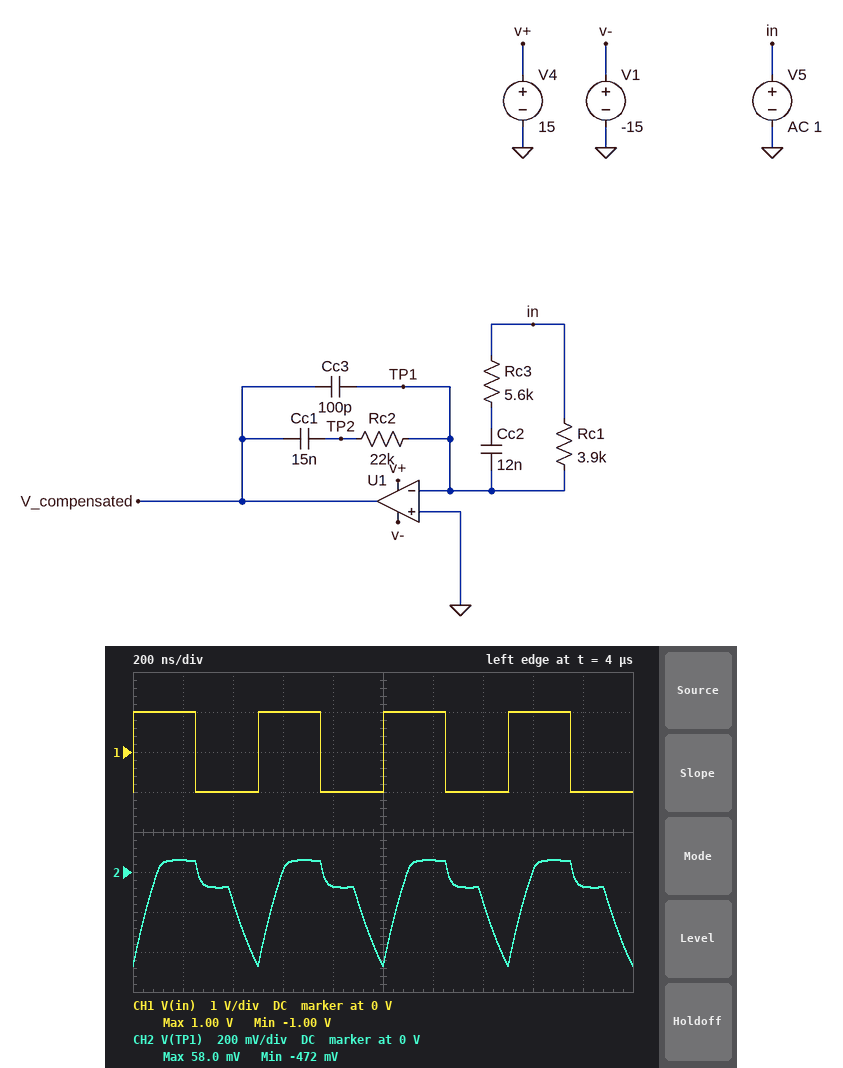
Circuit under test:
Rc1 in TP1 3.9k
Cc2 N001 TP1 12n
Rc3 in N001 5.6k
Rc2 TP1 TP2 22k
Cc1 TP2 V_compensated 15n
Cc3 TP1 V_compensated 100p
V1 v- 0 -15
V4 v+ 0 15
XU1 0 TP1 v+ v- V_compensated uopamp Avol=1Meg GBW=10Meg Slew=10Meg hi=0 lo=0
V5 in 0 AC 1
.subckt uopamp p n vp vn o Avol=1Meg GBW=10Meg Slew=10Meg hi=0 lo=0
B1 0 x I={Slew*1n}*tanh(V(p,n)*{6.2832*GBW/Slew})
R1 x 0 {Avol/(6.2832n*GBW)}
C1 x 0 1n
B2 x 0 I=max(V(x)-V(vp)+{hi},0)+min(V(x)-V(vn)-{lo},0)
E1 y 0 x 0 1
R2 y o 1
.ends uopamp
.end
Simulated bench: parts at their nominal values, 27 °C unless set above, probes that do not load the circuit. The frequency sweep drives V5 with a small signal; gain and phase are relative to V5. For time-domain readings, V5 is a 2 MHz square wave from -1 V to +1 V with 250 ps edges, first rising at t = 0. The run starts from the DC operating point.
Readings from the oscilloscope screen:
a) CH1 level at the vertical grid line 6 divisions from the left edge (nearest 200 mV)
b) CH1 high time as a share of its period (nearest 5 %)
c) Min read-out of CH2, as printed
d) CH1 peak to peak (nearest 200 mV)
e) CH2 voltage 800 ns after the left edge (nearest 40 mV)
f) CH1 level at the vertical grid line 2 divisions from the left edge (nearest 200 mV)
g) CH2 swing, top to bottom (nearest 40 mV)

1.0 V
50 %
-472 mV
2.0 V
-80 mV
-1.0 V
520 mV
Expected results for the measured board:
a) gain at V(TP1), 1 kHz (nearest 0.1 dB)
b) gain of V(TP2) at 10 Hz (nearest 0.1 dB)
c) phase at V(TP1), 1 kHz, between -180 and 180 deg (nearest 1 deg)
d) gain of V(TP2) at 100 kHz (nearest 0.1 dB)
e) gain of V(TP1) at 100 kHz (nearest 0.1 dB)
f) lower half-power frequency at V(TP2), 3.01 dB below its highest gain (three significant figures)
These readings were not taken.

-63.0 dB
15.0 dB
76 deg
14.6 dB
-25.4 dB
1.16 kHz
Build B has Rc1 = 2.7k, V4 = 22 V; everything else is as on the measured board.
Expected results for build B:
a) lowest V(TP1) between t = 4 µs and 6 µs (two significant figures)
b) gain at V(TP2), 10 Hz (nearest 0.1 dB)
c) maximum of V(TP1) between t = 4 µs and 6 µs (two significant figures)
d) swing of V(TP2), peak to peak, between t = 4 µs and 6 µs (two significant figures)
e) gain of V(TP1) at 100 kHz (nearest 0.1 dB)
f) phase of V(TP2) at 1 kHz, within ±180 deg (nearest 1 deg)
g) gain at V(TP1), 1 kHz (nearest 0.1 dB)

-490 mV
18.2 dB
76 mV
730 mV
-23.5 dB
-172 deg
-60.2 dB
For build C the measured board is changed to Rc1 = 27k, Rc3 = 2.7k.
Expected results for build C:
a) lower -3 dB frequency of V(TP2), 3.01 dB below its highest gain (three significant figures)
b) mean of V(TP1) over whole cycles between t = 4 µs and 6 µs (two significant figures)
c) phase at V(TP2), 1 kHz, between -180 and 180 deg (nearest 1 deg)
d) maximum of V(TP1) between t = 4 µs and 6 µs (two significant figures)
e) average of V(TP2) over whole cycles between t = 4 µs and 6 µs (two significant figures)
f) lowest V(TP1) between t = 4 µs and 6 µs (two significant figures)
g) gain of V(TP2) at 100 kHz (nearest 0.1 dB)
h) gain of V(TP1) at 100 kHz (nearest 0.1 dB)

4.30 kHz
-130 mV
-126 deg
53 mV
-1.1 V
-500 mV
14.0 dB
-26.0 dB
